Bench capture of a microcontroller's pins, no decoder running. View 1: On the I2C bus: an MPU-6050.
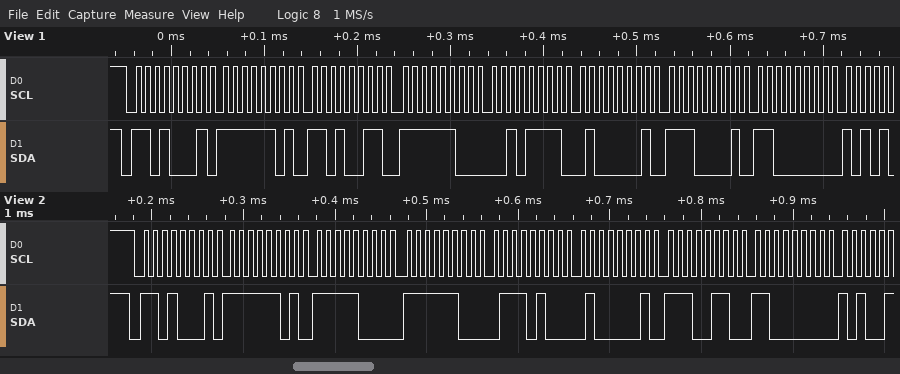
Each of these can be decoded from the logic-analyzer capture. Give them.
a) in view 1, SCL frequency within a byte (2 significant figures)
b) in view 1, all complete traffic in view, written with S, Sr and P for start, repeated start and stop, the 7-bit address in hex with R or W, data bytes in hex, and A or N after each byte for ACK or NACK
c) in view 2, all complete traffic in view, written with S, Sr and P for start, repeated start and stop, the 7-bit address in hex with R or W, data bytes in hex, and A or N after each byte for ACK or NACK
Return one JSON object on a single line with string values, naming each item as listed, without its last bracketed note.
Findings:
{"in view 1, SCL frequency within a byte": "100 kHz", "in view 1, all complete traffic in view, written with S, Sr and P for start, repeated start and stop, the 7-bit address in hex with R or W, data bytes in hex, and A or N after each byte for ACK or NACK": "S 68R A FD A D3 A FC A 2F A 41 A E1 A C0 A", "in view 2, all complete traffic in view, written with S, Sr and P for start, repeated start and stop, the 7-bit address in hex with R or W, data bytes in hex, and A or N after each byte for ACK or NACK": "S 68R A FD A F8 A FC A 74 A 41 A E6 A C0 A"}
